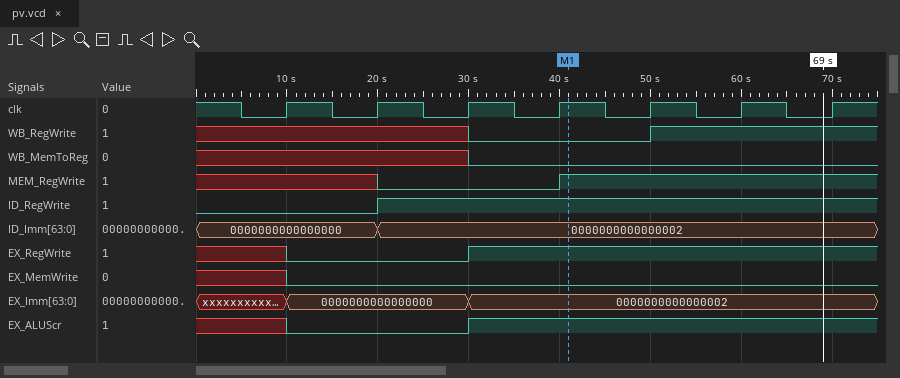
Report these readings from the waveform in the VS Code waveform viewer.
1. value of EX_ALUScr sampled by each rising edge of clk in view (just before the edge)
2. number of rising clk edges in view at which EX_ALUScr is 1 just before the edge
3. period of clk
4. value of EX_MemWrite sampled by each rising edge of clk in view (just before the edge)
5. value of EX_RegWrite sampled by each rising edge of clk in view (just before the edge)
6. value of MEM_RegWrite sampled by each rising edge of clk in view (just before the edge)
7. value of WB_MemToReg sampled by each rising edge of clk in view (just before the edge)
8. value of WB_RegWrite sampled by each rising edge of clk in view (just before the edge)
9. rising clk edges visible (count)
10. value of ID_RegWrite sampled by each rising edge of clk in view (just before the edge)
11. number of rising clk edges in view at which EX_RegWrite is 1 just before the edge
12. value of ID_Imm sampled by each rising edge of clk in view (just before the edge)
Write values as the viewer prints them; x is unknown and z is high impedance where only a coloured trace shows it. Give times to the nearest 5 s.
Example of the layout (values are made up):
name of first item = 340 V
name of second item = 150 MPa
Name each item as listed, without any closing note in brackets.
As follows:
value of EX_ALUScr sampled by each rising edge of clk in view = x 0 0 1 1 1 1
number of rising clk edges in view at which EX_ALUScr is 1 just before the edge = 4
period of clk = 10 s
value of EX_MemWrite sampled by each rising edge of clk in view = x 0 0 0 0 0 0
value of EX_RegWrite sampled by each rising edge of clk in view = x 0 0 1 1 1 1
value of MEM_RegWrite sampled by each rising edge of clk in view = x x 0 0 1 1 1
value of WB_MemToReg sampled by each rising edge of clk in view = x x x 0 0 0 0
value of WB_RegWrite sampled by each rising edge of clk in view = x x x 0 0 1 1
rising clk edges visible = 7
value of ID_RegWrite sampled by each rising edge of clk in view = 0 0 1 1 1 1 1
number of rising clk edges in view at which EX_RegWrite is 1 just before the edge = 4
value of ID_Imm sampled by each rising edge of clk in view = 0000000000000000, 0000000000000000, 0000000000000002, 0000000000000002, 0000000000000002, 0000000000000002, 0000000000000002
